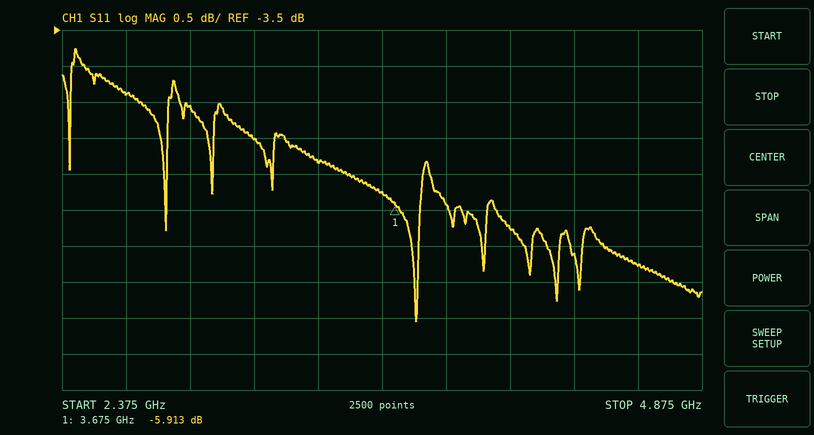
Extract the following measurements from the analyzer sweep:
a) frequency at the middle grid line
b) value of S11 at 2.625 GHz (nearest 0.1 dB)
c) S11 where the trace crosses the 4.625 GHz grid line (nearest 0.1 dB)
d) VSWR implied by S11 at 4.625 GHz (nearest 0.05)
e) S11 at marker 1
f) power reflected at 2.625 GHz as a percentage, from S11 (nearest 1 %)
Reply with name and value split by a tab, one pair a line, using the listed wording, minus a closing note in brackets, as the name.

frequency at the middle grid line	3.625 GHz
value of S11 at 2.625 GHz	-4.4 dB
S11 where the trace crosses the 4.625 GHz grid line	-6.8 dB
VSWR implied by S11 at 4.625 GHz	2.70
S11 at marker 1	-5.913 dB
power reflected at 2.625 GHz as a percentage, from S11	36 %
